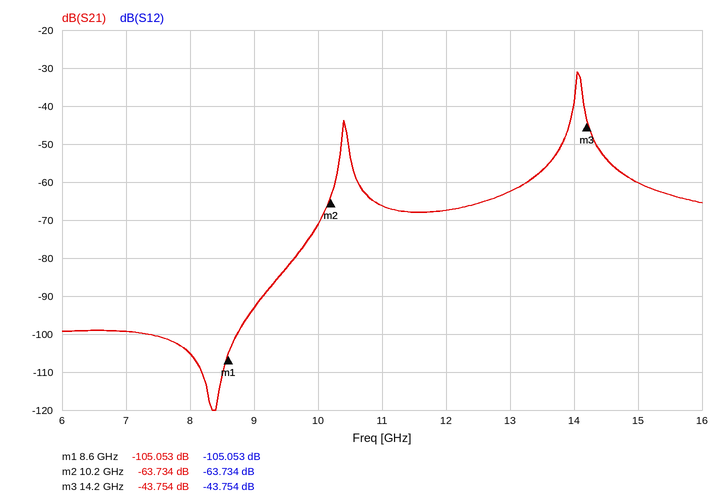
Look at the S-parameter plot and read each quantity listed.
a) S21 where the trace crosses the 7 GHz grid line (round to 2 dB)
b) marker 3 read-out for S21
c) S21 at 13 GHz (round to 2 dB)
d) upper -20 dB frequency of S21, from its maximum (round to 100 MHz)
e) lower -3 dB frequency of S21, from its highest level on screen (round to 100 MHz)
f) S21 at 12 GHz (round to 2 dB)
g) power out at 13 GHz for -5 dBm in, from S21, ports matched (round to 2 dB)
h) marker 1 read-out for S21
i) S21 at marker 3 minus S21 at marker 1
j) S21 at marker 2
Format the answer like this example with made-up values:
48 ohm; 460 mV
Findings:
-100 dB; -43.754 dB; -62 dB; 14.4 GHz; 14.0 GHz; -68 dB; -68 dBm; -105.053 dB; 61.299 dB; -63.734 dB
